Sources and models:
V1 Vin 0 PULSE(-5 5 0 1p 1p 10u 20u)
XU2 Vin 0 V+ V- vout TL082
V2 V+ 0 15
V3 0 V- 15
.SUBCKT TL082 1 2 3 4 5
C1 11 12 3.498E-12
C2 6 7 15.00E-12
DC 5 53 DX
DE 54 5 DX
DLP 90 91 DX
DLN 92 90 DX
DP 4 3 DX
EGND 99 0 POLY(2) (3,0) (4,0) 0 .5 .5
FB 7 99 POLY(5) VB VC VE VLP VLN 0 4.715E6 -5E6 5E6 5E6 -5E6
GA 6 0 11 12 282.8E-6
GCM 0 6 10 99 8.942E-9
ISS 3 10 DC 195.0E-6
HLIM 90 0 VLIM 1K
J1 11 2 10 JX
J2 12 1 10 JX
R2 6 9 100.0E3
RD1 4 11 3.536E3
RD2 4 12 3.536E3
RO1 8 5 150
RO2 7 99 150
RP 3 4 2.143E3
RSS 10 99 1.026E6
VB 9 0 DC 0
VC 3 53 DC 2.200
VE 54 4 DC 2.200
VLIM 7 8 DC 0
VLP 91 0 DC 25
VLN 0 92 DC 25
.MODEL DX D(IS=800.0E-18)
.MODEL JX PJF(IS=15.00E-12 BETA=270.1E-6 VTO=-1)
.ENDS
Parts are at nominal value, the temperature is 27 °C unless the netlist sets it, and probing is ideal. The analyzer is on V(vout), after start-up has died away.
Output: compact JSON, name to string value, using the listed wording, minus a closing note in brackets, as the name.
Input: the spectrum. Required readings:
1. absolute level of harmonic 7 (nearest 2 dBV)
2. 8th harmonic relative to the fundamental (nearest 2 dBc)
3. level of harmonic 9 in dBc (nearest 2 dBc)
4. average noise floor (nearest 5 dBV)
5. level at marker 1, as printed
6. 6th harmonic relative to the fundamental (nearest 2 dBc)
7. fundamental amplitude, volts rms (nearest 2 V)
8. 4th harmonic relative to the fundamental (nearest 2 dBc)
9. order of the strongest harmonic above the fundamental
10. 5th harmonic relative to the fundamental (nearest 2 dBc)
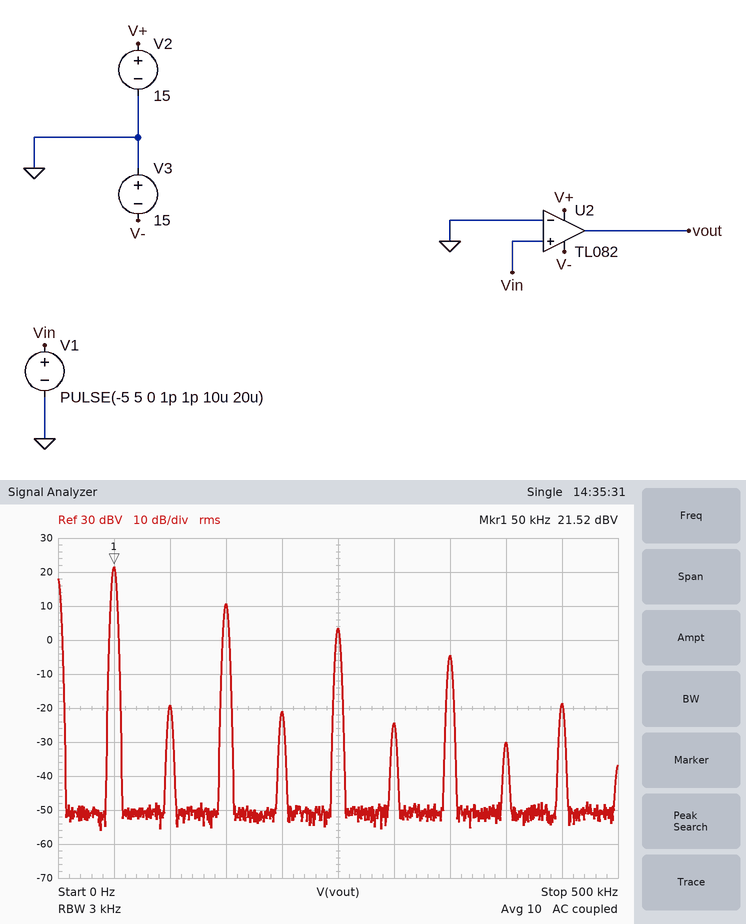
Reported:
{"absolute level of harmonic 7": "-4 dBV", "8th harmonic relative to the fundamental": "-52 dBc", "level of harmonic 9 in dBc": "-40 dBc", "average noise floor": "-50 dBV", "level at marker 1, as printed": "21.52 dBV", "6th harmonic relative to the fundamental": "-46 dBc", "fundamental amplitude, volts rms": "12 V", "4th harmonic relative to the fundamental": "-42 dBc", "order of the strongest harmonic above the fundamental": "3", "5th harmonic relative to the fundamental": "-18 dBc"}
